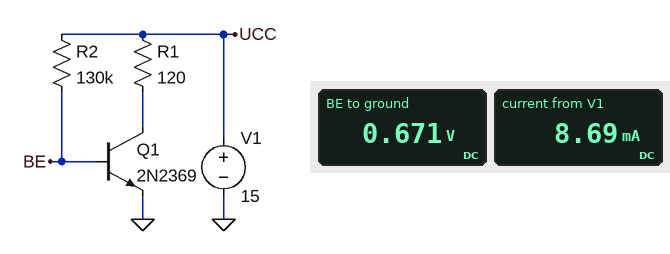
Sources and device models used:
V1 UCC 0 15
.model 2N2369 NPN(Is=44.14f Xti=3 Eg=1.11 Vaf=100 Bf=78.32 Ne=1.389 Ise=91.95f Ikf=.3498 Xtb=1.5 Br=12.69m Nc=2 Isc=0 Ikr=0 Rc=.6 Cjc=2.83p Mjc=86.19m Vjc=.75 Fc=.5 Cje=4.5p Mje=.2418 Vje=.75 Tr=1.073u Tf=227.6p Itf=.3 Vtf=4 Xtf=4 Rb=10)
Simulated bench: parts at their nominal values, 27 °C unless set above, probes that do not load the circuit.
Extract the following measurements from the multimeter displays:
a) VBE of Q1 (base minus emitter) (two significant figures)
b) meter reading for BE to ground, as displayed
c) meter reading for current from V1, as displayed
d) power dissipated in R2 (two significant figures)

670 mV
0.671 V
8.69 mA
1.6 mW
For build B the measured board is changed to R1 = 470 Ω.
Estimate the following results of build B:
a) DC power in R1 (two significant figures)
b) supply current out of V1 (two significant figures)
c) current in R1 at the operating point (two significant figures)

33 mW
8.5 mA
8.4 mA
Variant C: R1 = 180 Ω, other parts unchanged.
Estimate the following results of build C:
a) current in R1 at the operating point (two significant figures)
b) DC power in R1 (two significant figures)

8.5 mA
13 mW
